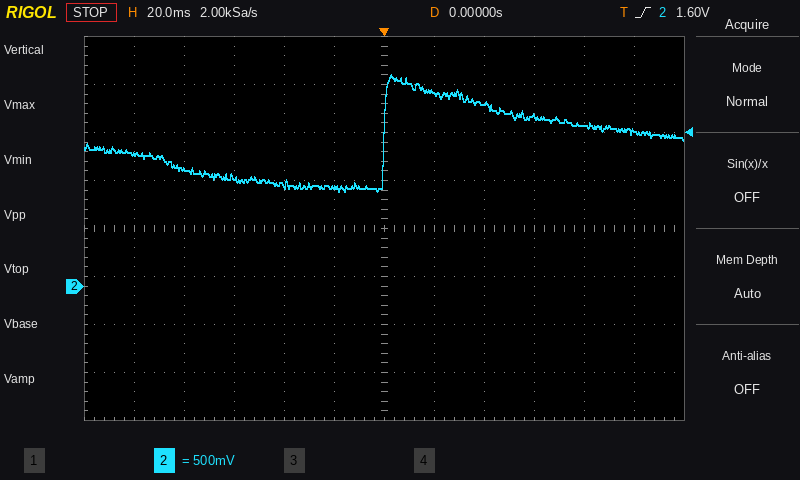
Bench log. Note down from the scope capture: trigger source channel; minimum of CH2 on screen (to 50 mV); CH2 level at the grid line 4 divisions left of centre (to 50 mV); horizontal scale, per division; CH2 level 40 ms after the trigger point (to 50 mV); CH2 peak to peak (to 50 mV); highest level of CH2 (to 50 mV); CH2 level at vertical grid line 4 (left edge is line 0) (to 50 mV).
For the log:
CH2
1.00 V
1.20 V
20 ms
1.90 V
1.20 V
2.20 V
1.05 V
